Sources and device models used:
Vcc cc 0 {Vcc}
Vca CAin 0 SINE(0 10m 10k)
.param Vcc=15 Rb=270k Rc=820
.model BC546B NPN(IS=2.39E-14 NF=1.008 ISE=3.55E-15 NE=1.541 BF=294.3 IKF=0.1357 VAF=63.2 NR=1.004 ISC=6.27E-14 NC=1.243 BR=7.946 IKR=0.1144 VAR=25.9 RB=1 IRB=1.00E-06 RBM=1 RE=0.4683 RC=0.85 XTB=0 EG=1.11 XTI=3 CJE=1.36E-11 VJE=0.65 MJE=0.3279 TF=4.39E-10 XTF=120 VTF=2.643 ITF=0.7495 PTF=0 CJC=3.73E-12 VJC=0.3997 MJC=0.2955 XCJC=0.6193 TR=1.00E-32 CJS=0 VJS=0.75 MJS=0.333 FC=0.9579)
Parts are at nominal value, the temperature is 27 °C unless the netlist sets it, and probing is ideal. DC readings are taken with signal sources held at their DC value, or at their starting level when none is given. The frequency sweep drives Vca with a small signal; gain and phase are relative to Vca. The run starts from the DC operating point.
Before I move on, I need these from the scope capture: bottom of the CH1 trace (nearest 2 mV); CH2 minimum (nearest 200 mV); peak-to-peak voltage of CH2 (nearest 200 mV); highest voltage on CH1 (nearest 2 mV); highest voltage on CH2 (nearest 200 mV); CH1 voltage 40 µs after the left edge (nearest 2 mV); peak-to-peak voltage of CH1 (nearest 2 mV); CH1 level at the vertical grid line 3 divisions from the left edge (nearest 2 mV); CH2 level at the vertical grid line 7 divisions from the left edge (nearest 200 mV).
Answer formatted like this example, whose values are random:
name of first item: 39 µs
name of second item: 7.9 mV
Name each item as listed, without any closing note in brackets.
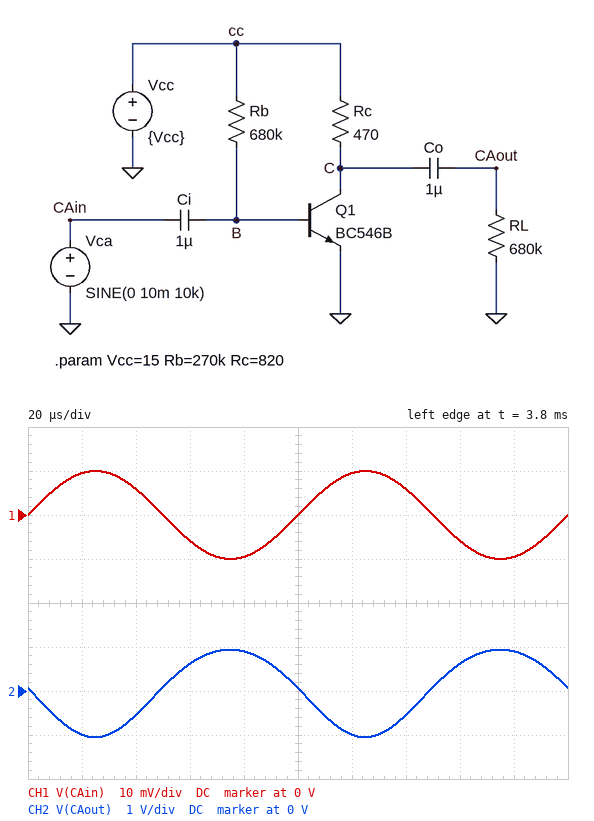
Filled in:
bottom of the CH1 trace: -10 mV
CH2 minimum: -1.0 V
peak-to-peak voltage of CH2: 2.0 V
highest voltage on CH1: 10 mV
highest voltage on CH2: 1.0 V
CH1 voltage 40 µs after the left edge: 6 mV
peak-to-peak voltage of CH1: 20 mV
CH1 level at the vertical grid line 3 divisions from the left edge: -6 mV
CH2 level at the vertical grid line 7 divisions from the left edge: -600 mV
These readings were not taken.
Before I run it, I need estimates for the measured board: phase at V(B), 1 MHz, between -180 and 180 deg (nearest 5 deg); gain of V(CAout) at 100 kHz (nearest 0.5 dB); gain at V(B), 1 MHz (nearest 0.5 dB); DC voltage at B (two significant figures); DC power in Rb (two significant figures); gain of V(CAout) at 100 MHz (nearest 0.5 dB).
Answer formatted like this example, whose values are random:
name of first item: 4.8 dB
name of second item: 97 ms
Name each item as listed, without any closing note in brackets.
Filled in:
phase at V(B), 1 MHz, between -180 and 180 deg: 0 deg
gain of V(CAout) at 100 kHz: 40.0 dB
gain at V(B), 1 MHz: 0 dB
DC voltage at B: 690 mV
DC power in Rb: 300 µW
gain of V(CAout) at 100 MHz: 39.0 dB
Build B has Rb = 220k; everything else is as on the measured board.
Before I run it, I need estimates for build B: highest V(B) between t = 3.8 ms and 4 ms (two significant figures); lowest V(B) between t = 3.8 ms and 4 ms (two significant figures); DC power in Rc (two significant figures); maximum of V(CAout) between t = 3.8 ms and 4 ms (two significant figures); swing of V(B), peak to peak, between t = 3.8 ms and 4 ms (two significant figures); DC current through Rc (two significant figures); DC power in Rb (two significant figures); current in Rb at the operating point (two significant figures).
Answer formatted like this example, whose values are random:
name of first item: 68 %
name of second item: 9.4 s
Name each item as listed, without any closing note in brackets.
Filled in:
highest V(B) between t = 3.8 ms and 4 ms: 730 mV
lowest V(B) between t = 3.8 ms and 4 ms: 710 mV
DC power in Rc: 150 mW
maximum of V(CAout) between t = 3.8 ms and 4 ms: 2.0 V
swing of V(B), peak to peak, between t = 3.8 ms and 4 ms: 20 mV
DC current through Rc: 18 mA
DC power in Rb: 930 µW
current in Rb at the operating point: 65 µA
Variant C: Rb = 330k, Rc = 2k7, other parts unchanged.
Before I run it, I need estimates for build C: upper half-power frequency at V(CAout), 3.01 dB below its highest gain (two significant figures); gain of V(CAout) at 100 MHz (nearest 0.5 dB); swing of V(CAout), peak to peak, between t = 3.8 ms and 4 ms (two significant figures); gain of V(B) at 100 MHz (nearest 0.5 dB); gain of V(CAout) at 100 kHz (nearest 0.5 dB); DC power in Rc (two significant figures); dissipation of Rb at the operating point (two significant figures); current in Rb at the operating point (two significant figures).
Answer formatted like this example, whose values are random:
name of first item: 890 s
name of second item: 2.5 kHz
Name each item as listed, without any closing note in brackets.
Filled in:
upper half-power frequency at V(CAout), 3.01 dB below its highest gain: 20 MHz
gain of V(CAout) at 100 MHz: 15.5 dB
swing of V(CAout), peak to peak, between t = 3.8 ms and 4 ms: 5.4 V
gain of V(B) at 100 MHz: 0 dB
gain of V(CAout) at 100 kHz: 29.5 dB
DC power in Rc: 82 mW
dissipation of Rb at the operating point: 620 µW
current in Rb at the operating point: 43 µA
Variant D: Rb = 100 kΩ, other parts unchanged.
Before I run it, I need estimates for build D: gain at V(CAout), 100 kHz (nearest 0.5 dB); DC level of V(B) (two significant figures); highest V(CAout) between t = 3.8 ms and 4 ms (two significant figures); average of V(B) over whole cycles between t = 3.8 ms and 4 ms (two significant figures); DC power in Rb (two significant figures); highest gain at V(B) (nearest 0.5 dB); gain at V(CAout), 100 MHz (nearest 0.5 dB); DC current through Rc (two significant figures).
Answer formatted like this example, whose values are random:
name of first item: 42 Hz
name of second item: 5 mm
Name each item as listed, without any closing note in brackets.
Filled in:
gain at V(CAout), 100 kHz: 46.0 dB
DC level of V(B): 750 mV
highest V(CAout) between t = 3.8 ms and 4 ms: 4.4 V
average of V(B) over whole cycles between t = 3.8 ms and 4 ms: 740 mV
DC power in Rb: 2.0 mW
highest gain at V(B): 0 dB
gain at V(CAout), 100 MHz: 25.5 dB
DC current through Rc: 31 mA
